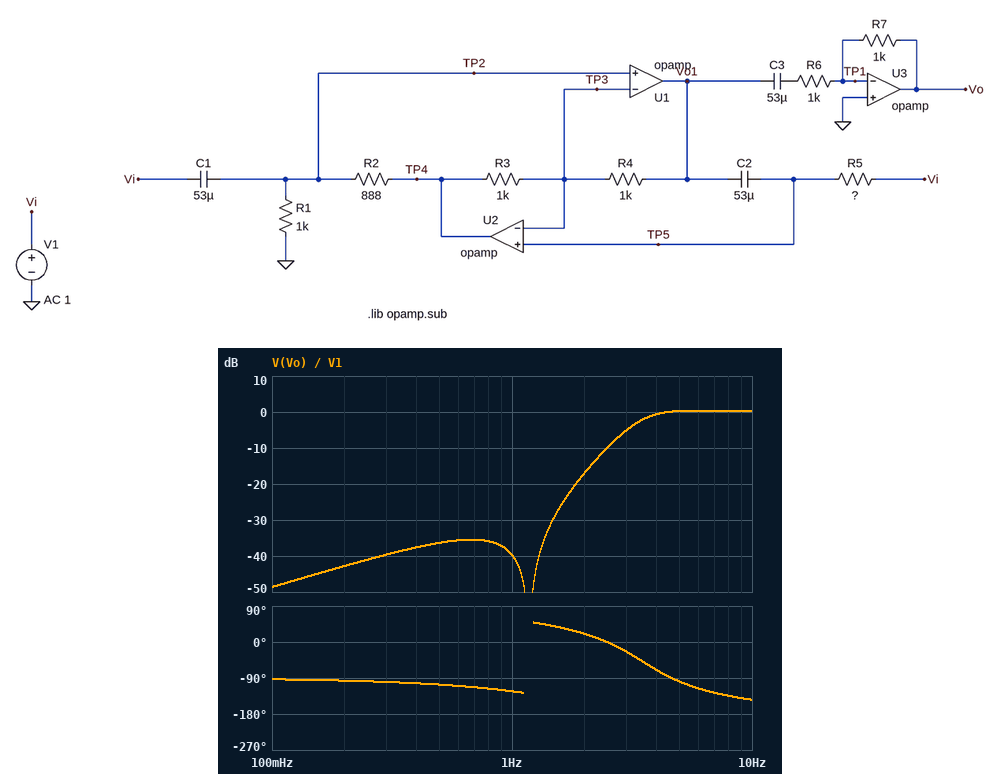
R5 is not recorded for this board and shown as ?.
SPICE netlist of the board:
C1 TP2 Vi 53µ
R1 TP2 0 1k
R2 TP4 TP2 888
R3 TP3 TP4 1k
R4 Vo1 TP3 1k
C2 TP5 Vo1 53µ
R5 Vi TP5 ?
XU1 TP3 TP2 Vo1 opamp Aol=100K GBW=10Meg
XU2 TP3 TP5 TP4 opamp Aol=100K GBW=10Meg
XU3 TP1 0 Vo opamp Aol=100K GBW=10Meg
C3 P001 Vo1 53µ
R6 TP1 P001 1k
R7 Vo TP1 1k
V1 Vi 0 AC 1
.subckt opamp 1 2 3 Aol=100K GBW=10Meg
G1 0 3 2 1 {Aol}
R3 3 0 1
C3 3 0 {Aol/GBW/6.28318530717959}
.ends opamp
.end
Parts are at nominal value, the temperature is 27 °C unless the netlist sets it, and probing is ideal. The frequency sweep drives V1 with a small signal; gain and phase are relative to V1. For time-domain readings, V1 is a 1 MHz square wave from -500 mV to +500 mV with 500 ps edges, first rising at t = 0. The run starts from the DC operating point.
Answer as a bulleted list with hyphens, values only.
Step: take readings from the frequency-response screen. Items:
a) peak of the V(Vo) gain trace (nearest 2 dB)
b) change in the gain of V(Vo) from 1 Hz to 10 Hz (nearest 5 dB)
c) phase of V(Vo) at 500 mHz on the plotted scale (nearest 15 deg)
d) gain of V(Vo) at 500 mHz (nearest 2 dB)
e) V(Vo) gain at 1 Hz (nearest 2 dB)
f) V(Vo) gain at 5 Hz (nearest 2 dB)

- 0 dB
- 40 dB
- -105 deg
- -36 dB
- -40 dB
- 0 dB
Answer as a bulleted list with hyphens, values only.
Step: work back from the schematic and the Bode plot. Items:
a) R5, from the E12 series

- 820 Ω
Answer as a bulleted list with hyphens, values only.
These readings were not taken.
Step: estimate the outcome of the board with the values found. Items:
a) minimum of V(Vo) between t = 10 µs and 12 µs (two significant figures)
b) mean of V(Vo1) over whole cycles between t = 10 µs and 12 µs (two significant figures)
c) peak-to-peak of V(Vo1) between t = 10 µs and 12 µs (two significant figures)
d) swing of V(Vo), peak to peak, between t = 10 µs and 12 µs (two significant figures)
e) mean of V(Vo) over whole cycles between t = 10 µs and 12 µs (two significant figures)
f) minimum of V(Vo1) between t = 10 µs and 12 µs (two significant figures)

- -1.0 V
- 440 mV
- 1.4 V
- 1.1 V
- -500 mV
- -260 mV
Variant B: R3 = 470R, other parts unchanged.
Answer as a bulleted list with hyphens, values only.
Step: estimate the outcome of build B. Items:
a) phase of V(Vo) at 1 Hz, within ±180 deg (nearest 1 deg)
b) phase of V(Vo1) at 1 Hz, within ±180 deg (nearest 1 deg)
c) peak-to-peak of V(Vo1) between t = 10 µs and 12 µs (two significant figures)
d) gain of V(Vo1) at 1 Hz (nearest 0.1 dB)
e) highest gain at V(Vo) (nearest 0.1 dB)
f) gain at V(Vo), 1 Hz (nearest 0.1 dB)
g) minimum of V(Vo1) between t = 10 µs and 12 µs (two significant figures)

- 40 deg
- 148 deg
- 1.5 V
- 0.7 dB
- 0.6 dB
- -9.3 dB
- 200 mV
